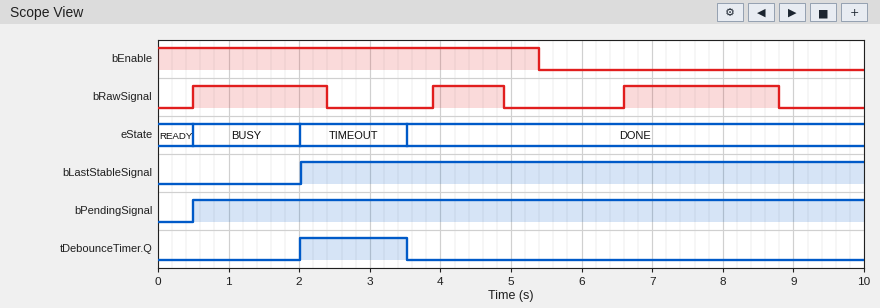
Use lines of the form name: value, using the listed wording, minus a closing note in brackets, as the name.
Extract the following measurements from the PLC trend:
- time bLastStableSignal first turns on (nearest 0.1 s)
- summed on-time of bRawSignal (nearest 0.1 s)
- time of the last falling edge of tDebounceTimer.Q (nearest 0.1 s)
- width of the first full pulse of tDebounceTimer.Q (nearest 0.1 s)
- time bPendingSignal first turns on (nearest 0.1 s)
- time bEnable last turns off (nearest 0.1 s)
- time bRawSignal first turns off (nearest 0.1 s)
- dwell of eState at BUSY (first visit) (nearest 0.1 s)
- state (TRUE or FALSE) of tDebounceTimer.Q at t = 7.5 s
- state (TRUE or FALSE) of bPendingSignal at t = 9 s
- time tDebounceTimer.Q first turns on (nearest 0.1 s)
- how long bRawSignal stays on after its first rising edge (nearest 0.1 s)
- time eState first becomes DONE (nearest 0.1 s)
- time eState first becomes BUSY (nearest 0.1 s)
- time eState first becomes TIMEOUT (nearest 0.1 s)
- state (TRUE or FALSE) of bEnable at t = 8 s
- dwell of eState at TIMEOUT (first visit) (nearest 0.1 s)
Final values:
time bLastStableSignal first turns on: 2.0 s
summed on-time of bRawSignal: 5.1 s
time of the last falling edge of tDebounceTimer.Q: 3.5 s
width of the first full pulse of tDebounceTimer.Q: 1.5 s
time bPendingSignal first turns on: 0.5 s
time bEnable last turns off: 5.4 s
time bRawSignal first turns off: 2.4 s
dwell of eState at BUSY (first visit): 1.5 s
state (TRUE or FALSE) of tDebounceTimer.Q at t = 7.5 s: FALSE
state (TRUE or FALSE) of bPendingSignal at t = 9 s: TRUE
time tDebounceTimer.Q first turns on: 2.0 s
how long bRawSignal stays on after its first rising edge: 1.9 s
time eState first becomes DONE: 3.5 s
time eState first becomes BUSY: 0.5 s
time eState first becomes TIMEOUT: 2.0 s
state (TRUE or FALSE) of bEnable at t = 8 s: FALSE
dwell of eState at TIMEOUT (first visit): 1.5 s
